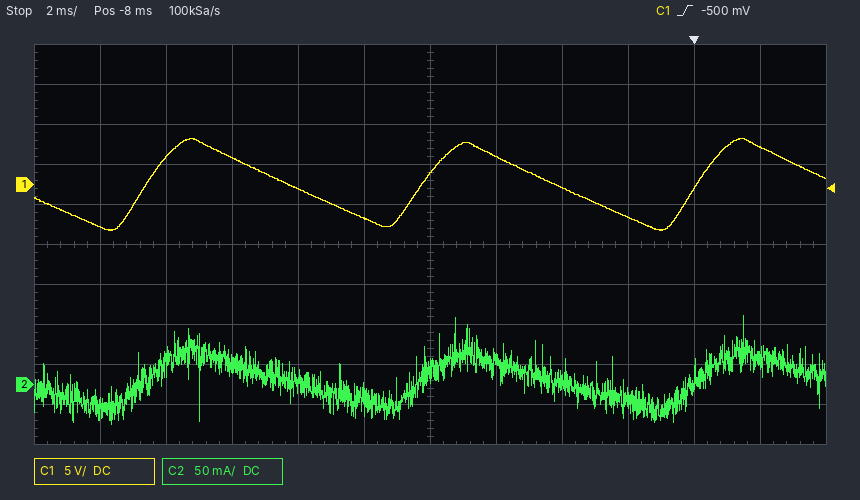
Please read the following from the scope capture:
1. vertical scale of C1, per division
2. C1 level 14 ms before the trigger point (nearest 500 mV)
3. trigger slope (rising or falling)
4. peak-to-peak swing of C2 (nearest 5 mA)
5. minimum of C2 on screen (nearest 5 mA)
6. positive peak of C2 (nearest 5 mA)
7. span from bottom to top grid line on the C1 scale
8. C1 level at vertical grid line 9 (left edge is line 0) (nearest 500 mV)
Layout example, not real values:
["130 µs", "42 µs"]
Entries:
["5 V", "3.5 V", "rising", "135 mA", "-50 mA", "85 mA", "50 V", "-4.0 V"]
